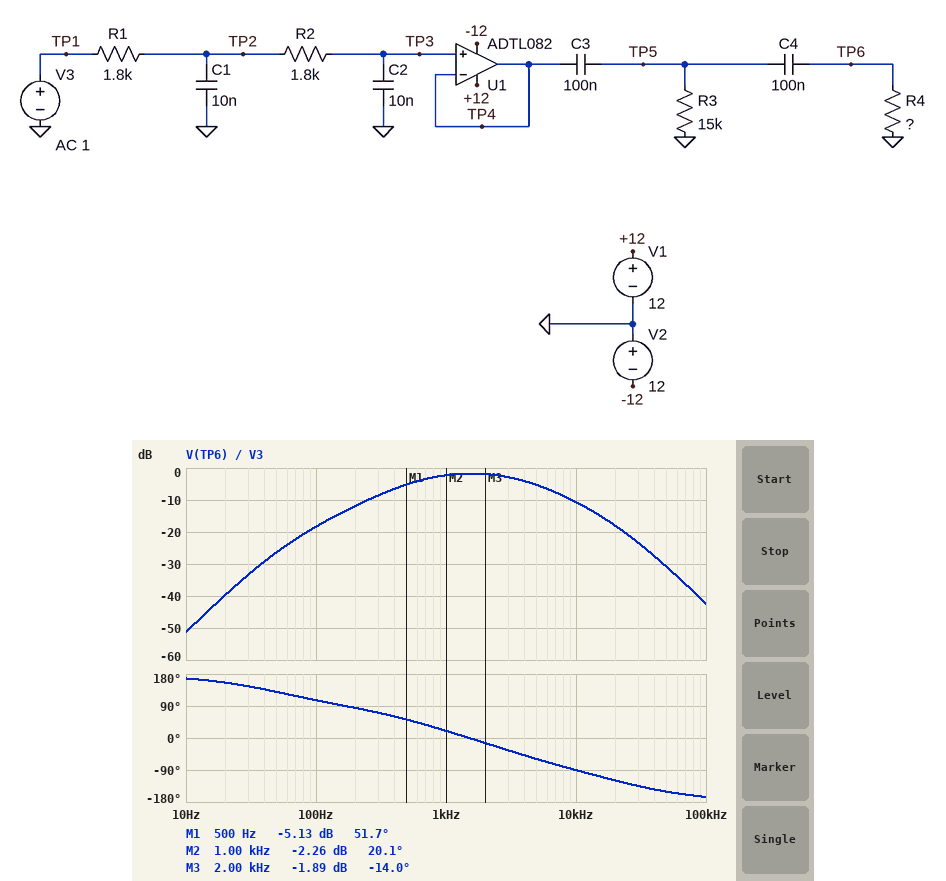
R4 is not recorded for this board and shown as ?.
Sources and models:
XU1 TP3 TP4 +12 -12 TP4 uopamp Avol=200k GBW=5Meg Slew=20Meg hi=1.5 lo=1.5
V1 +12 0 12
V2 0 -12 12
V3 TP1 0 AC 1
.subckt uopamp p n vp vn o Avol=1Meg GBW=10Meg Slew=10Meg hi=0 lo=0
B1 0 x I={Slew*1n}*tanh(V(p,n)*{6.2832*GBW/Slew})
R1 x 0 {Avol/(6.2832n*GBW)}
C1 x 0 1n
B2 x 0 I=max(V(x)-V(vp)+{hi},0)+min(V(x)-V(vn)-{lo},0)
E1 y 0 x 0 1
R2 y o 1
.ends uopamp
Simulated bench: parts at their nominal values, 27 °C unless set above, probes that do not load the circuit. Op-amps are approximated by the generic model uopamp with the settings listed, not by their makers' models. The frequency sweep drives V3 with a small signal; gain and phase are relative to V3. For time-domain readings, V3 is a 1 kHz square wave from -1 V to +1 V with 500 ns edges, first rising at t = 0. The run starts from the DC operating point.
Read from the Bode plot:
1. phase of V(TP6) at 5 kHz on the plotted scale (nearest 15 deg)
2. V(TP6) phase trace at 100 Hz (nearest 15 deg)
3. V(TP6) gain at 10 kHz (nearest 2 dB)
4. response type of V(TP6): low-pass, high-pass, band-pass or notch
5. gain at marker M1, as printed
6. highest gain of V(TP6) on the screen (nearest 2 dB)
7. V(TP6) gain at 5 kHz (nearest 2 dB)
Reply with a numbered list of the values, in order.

1. -60 deg
2. 105 deg
3. -10 dB
4. band-pass
5. -5.13 dB
6. -2 dB
7. -6 dB
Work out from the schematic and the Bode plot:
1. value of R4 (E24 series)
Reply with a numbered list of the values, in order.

1. 4.7 kΩ
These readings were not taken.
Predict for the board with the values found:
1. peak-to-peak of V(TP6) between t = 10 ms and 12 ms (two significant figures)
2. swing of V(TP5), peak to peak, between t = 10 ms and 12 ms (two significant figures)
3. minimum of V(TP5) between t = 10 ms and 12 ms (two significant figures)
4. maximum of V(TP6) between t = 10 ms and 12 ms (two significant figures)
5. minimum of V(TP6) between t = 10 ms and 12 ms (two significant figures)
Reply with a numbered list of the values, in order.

1. 2.4 V
2. 2.1 V
3. -1.0 V
4. 1.2 V
5. -1.2 V
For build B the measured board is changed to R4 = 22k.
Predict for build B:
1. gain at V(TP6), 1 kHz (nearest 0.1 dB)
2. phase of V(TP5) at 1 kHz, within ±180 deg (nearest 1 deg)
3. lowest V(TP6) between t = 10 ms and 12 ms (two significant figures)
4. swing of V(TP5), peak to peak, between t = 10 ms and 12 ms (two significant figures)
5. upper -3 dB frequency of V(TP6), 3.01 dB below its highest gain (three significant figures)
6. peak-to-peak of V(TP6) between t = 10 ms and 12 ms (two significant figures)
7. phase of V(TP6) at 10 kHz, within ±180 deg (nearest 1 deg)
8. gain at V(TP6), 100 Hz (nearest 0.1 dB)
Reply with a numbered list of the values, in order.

1. -0.6 dB
2. -9 deg
3. -1.1 V
4. 2.1 V
5. 3.71 kHz
6. 2.2 V
7. -93 deg
8. -8.0 dB
